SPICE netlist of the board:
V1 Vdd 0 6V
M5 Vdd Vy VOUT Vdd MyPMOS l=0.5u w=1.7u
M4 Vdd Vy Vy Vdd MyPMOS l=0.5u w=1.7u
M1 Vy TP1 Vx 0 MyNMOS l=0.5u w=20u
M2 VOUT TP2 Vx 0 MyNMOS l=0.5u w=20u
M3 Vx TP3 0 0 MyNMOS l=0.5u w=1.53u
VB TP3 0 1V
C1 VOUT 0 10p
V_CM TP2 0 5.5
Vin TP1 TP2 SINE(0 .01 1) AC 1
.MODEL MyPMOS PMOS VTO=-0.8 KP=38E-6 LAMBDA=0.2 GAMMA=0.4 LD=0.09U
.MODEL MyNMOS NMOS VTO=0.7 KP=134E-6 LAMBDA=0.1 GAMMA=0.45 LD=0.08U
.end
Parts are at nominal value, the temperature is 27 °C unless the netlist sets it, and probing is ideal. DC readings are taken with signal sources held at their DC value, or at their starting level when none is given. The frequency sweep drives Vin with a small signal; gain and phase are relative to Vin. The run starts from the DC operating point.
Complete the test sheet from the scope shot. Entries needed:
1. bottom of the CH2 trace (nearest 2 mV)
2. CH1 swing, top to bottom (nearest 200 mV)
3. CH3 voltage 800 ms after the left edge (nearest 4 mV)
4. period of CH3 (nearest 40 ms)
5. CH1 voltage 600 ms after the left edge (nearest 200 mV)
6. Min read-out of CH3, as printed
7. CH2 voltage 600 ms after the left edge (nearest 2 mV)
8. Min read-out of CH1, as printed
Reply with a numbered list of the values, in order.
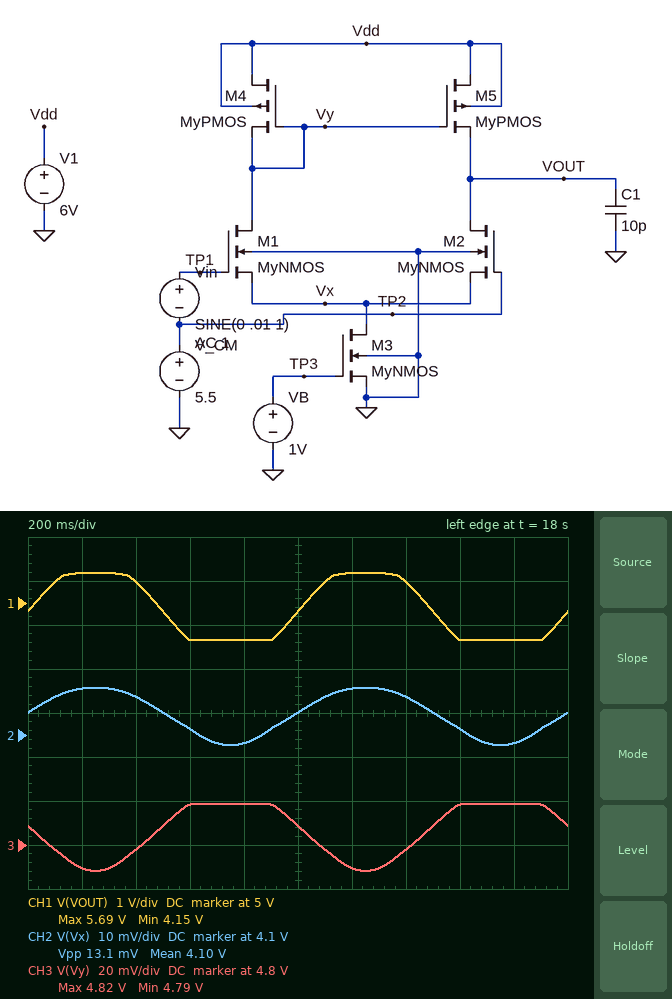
1. 4.098 V
2. 1.6 V
3. 4.820 V
4. 1.00 s
5. 4.2 V
6. 4.79 V
7. 4.102 V
8. 4.15 V
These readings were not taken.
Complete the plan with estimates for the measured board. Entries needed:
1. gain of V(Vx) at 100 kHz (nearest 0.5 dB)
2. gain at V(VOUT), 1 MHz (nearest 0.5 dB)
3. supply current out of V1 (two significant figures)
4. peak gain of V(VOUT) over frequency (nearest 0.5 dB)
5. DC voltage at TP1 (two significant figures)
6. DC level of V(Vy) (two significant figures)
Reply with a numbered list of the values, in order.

1. -6.0 dB
2. 19.0 dB
3. 38 µA
4. 41.0 dB
5. 5.5 V
6. 4.8 V
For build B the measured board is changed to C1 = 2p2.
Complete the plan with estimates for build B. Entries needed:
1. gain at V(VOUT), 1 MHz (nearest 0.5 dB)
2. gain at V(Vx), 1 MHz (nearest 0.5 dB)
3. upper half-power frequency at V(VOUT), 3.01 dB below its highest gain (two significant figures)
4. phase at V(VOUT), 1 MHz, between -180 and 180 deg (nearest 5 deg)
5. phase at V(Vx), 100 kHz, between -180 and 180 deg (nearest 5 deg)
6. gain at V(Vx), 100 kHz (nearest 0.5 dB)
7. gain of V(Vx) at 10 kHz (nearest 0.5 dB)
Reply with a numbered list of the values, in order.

1. 31.5 dB
2. -6.5 dB
3. 350 kHz
4. -70 deg
5. -5 deg
6. -4.5 dB
7. -4.5 dB
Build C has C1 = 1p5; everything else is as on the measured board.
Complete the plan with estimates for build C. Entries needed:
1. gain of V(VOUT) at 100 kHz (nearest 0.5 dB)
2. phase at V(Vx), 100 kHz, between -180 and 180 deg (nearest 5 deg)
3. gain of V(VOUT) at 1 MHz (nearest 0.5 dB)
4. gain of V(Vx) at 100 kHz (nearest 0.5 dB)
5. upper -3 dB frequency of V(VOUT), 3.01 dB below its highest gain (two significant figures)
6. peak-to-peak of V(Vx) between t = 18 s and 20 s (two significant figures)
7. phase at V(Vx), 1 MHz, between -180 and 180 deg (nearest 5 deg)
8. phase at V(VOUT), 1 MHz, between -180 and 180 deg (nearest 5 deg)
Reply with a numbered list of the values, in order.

1. 41.0 dB
2. -5 deg
3. 34.5 dB
4. -4.5 dB
5. 510 kHz
6. 13 mV
7. -10 deg
8. -65 deg
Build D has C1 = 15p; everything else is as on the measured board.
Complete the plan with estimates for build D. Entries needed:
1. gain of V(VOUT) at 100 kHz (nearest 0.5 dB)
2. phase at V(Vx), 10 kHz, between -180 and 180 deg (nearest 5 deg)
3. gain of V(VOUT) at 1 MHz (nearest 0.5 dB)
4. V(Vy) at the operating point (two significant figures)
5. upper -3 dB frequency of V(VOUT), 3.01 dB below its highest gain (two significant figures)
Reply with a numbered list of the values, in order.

1. 34.5 dB
2. -5 deg
3. 15.5 dB
4. 4.8 V
5. 51 kHz
